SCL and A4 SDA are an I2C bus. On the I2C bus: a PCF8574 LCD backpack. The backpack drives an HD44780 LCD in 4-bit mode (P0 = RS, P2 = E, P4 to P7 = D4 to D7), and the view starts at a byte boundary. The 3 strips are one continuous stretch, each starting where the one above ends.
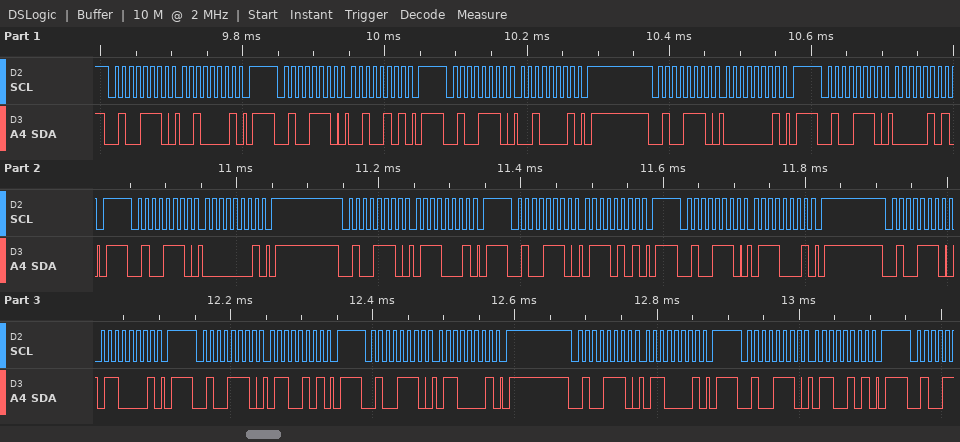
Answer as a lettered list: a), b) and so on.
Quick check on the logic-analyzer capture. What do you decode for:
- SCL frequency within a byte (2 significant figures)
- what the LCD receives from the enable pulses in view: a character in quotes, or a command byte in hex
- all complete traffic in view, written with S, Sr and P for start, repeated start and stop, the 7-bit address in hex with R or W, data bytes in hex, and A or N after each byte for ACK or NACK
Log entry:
a) 100 kHz
b) ' ' 'v'
c) S 27W A 21 A P S 27W A 25 A P S 27W A 21 A P S 27W A 01 A P S 27W A 05 A P S 27W A 01 A P S 27W A 71 A P S 27W A 75 A P S 27W A 71 A P S 27W A 61 A P S 27W A 65 A P S 27W A 61 A P S 27W A 61 A P S 27W A 65 A P
